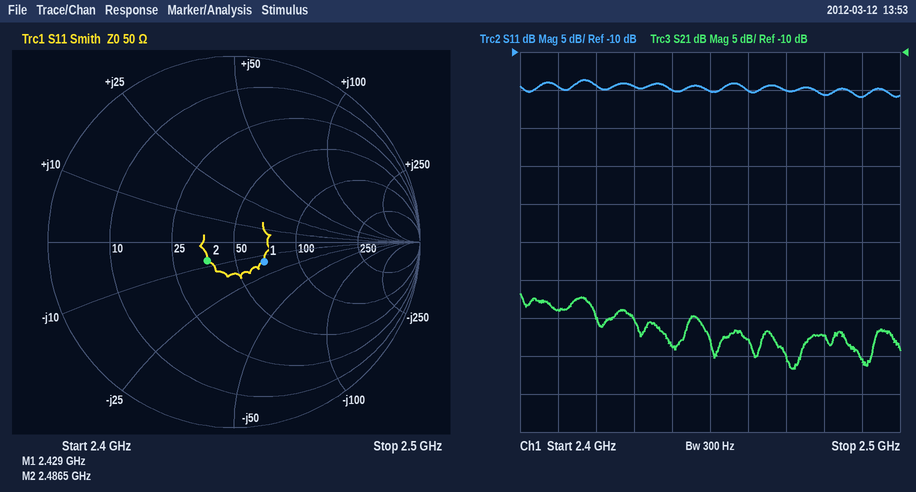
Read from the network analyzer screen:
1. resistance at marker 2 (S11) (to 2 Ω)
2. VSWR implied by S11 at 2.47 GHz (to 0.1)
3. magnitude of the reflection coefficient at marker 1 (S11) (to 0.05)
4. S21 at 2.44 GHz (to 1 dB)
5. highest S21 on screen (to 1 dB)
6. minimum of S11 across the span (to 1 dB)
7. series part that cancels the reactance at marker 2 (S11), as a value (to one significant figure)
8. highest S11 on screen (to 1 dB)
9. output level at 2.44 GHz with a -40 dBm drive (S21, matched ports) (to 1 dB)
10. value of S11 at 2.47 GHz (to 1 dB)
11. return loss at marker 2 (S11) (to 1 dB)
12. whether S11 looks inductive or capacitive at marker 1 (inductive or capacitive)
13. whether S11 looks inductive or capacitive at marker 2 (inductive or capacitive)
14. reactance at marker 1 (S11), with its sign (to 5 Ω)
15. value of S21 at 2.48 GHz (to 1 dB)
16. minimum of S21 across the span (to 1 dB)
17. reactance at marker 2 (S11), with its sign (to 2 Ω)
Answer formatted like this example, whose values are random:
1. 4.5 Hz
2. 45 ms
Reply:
1. 36 Ω
2. 1.4
3. 0.20
4. -49 dB
5. -42 dB
6. -16 dB
7. 500 pH
8. -14 dB
9. -89 dBm
10. -15 dB
11. 15 dB
12. capacitive
13. capacitive
14. -15 Ω
15. -47 dB
16. -52 dB
17. -8 Ω
